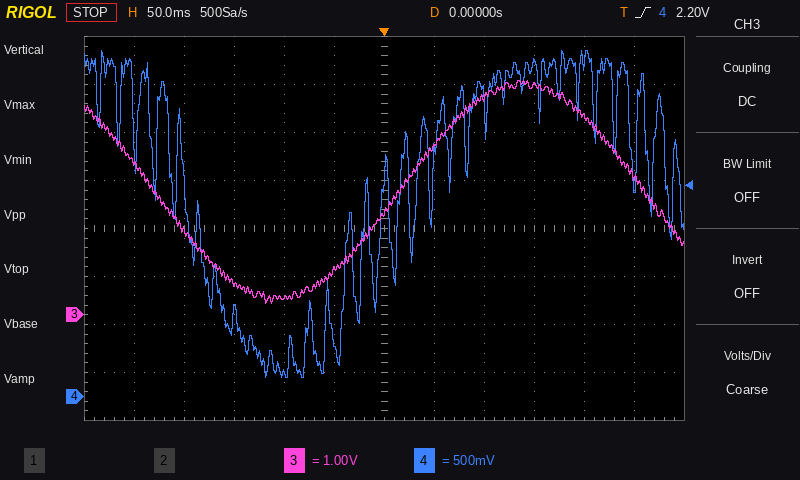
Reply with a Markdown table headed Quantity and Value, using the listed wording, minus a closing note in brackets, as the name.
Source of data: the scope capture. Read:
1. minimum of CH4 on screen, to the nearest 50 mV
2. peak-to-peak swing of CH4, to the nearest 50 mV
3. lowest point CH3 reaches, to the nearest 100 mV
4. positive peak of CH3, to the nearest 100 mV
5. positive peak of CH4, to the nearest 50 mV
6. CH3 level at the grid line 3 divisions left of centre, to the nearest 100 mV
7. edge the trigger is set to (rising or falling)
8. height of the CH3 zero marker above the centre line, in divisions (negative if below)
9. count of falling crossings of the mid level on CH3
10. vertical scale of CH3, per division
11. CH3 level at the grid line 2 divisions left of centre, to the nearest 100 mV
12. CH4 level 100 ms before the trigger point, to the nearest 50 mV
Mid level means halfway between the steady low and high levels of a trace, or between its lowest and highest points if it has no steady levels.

| Quantity | Value |
|---|---|
| minimum of CH4 on screen, to the nearest 50 mV | 200 mV |
| peak-to-peak swing of CH4, to the nearest 50 mV | 3.40 V |
| lowest point CH3 reaches, to the nearest 100 mV | 200 mV |
| positive peak of CH3, to the nearest 100 mV | 4.9 V |
| positive peak of CH4, to the nearest 50 mV | 3.60 V |
| CH3 level at the grid line 3 divisions left of centre, to the nearest 100 mV | 700 mV |
| edge the trigger is set to | rising |
| height of the CH3 zero marker above the centre line, in divisions | -1.8 div |
| count of falling crossings of the mid level on CH3 | 2 |
| vertical scale of CH3, per division | 1 V |
| CH3 level at the grid line 2 divisions left of centre, to the nearest 100 mV | 400 mV |
| CH4 level 100 ms before the trigger point, to the nearest 50 mV | 250 mV |
